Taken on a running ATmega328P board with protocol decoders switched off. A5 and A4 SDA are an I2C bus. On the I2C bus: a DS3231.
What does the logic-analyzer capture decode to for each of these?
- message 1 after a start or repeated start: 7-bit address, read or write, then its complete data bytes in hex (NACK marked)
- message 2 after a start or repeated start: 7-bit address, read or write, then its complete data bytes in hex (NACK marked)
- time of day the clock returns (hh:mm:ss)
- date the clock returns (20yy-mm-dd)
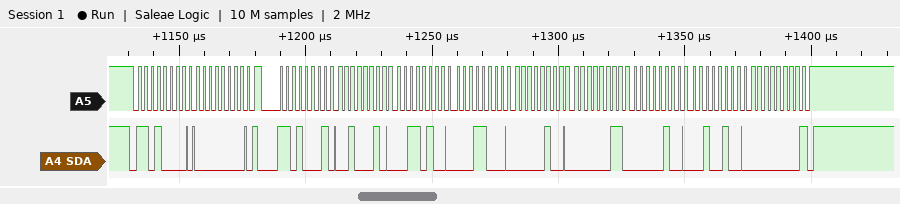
0x68 write: 00
0x68 read: 22 34 18 04 03 04 24 00 NACK
18:34:22
2024-04-03
